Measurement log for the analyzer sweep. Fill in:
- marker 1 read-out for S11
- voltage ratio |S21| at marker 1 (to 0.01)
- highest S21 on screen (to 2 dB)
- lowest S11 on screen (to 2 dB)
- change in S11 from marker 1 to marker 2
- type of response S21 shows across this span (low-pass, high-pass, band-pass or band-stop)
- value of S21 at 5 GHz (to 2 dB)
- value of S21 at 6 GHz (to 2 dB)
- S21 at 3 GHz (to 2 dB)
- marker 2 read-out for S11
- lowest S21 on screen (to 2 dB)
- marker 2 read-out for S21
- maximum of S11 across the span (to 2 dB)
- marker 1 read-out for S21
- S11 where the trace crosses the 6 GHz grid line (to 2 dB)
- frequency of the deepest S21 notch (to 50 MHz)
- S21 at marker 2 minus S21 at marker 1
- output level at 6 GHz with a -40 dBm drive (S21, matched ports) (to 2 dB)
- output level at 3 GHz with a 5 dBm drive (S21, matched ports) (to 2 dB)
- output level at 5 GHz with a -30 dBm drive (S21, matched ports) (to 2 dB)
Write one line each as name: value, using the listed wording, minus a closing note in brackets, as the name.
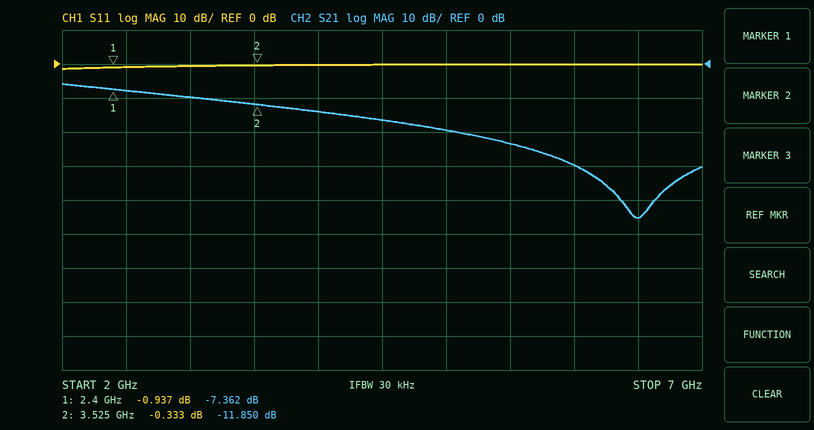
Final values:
marker 1 read-out for S11: -0.937 dB
voltage ratio |S21| at marker 1: 0.43
highest S21 on screen: -6 dB
lowest S11 on screen: -2 dB
change in S11 from marker 1 to marker 2: 0.604 dB
type of response S21 shows across this span: low-pass
value of S21 at 5 GHz: -20 dB
value of S21 at 6 GHz: -30 dB
S21 at 3 GHz: -10 dB
marker 2 read-out for S11: -0.333 dB
lowest S21 on screen: -46 dB
marker 2 read-out for S21: -11.850 dB
maximum of S11 across the span: 0 dB
marker 1 read-out for S21: -7.362 dB
S11 where the trace crosses the 6 GHz grid line: 0 dB
frequency of the deepest S21 notch: 6.50 GHz
S21 at marker 2 minus S21 at marker 1: -4.488 dB
output level at 6 GHz with a -40 dBm drive (S21, matched ports): -70 dBm
output level at 3 GHz with a 5 dBm drive (S21, matched ports): -4 dBm
output level at 5 GHz with a -30 dBm drive (S21, matched ports): -50 dBm
